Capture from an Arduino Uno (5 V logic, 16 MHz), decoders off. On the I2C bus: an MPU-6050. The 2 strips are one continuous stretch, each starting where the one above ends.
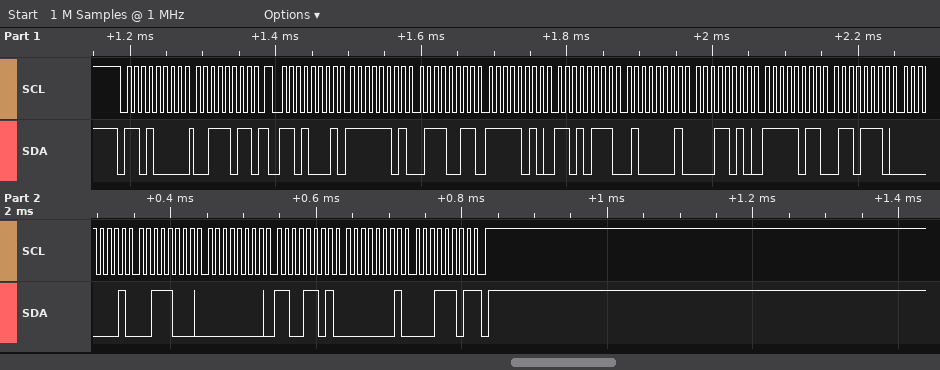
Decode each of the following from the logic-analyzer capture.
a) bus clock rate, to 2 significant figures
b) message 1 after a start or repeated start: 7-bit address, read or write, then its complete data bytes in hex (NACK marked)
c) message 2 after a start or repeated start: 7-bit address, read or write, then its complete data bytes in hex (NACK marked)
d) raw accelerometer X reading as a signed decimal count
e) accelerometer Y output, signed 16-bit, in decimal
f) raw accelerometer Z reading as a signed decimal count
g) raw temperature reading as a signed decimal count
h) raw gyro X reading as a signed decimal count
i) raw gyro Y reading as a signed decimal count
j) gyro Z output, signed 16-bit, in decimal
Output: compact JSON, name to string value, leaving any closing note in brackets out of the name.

{"bus clock rate, to 2 significant figures": "100 kHz", "message 1 after a start or repeated start: 7-bit address, read or write, then its complete data bytes in hex": "0x68 write: 3B", "message 2 after a start or repeated start: 7-bit address, read or write, then its complete data bytes in hex": "0x68 read: FD 73 FA D7 41 1A FB 6E 01 38 00 CD 01 1D NACK", "raw accelerometer X reading as a signed decimal count": "-653", "accelerometer Y output, signed 16-bit, in decimal": "-1321", "raw accelerometer Z reading as a signed decimal count": "16666", "raw temperature reading as a signed decimal count": "-1170", "raw gyro X reading as a signed decimal count": "312", "raw gyro Y reading as a signed decimal count": "205", "gyro Z output, signed 16-bit, in decimal": "285"}
